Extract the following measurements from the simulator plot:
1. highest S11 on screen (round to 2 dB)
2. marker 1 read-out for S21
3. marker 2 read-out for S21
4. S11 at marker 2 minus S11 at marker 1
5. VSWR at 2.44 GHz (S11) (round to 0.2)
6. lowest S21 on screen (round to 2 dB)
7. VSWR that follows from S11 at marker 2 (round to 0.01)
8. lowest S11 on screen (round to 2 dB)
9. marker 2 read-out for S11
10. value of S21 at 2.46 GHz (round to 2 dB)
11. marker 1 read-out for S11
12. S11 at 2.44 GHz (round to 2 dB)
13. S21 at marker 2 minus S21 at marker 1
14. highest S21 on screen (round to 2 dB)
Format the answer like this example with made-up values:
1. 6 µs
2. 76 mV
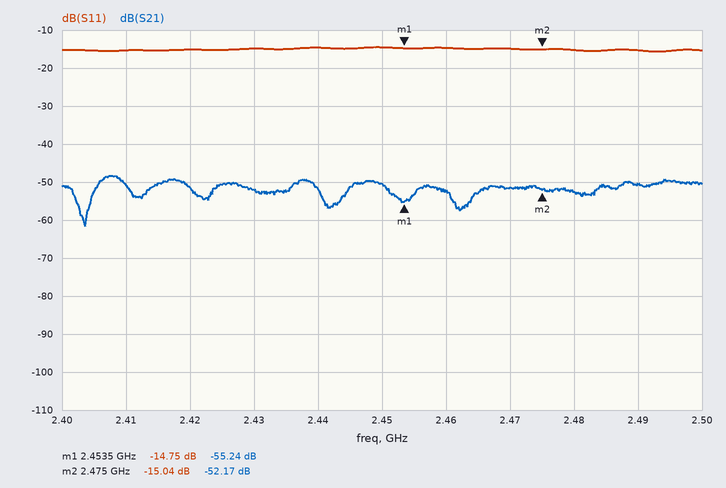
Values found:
1. -14 dB
2. -55.24 dB
3. -52.17 dB
4. -0.29 dB
5. 1.4
6. -62 dB
7. 1.43
8. -16 dB
9. -15.04 dB
10. -52 dB
11. -14.75 dB
12. -14 dB
13. 3.07 dB
14. -48 dB
